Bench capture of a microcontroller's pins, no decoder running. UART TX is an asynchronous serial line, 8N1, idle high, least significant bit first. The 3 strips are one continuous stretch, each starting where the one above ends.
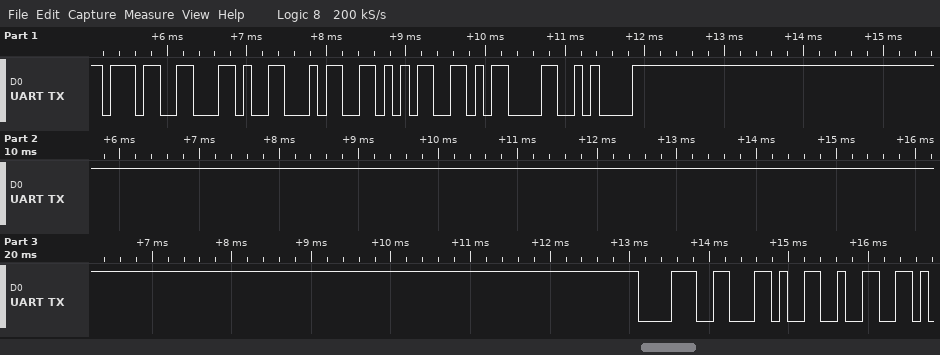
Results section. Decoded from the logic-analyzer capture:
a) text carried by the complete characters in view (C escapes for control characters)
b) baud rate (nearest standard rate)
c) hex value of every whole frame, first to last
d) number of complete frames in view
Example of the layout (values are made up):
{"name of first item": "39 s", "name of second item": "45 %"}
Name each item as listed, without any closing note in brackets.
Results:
{"text carried by the complete characters in view": "\"7,45\\r\\n8,2\"", "baud rate": "9600 baud", "hex value of every whole frame, first to last": "0x37 0x2C 0x34 0x35 0x0D 0x0A 0x38 0x2C 0x32", "number of complete frames in view": "9"}
